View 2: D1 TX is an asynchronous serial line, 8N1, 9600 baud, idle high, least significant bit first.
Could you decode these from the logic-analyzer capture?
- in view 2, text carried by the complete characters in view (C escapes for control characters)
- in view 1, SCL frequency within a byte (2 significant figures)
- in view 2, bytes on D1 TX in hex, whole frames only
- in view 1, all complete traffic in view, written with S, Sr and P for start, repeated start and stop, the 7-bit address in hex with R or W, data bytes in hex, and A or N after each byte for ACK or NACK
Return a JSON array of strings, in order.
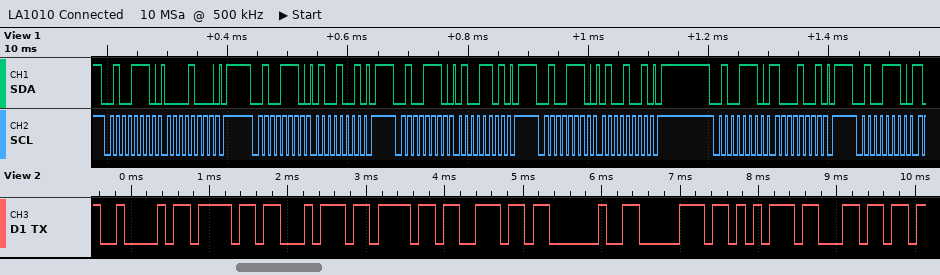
["\"Boton pul\"", "100 kHz", "0x42 0x6F 0x74 0x6F 0x6E 0x20 0x70 0x75 0x6C", "S 27W A 08 A P S 27W A 49 A P S 27W A 4D A P S 27W A 49 A P S 27W A 89 A P S 27W A"]
